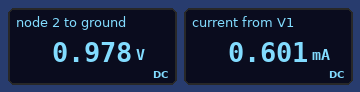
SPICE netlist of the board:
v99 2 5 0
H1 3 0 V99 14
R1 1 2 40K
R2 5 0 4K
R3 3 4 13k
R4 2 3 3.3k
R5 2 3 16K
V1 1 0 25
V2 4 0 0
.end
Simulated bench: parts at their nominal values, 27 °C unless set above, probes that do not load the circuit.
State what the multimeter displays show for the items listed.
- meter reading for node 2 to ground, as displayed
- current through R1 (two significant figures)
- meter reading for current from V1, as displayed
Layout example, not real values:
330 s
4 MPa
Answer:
0.978 V
600 µA
0.601 mA
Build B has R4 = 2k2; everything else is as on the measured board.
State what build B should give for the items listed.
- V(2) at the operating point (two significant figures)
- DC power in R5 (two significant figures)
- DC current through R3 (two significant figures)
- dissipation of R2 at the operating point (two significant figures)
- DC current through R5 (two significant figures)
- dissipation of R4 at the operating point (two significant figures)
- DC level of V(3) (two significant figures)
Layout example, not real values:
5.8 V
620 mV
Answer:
790 mV
39 µW
210 nA
160 µW
49 µA
280 µW
2.8 mV
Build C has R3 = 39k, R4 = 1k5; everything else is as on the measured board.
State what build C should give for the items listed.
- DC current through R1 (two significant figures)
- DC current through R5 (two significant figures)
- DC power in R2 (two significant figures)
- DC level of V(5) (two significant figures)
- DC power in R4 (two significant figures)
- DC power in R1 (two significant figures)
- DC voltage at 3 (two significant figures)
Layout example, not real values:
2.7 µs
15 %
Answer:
610 µA
39 µA
97 µW
620 mV
260 µW
15 mW
2.2 mV
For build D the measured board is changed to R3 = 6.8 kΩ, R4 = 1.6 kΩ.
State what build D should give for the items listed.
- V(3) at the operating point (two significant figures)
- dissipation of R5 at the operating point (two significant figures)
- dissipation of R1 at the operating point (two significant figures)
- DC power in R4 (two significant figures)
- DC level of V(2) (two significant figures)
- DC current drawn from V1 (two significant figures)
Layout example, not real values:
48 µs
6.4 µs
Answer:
2.3 mV
26 µW
15 mW
260 µW
650 mV
610 µA
